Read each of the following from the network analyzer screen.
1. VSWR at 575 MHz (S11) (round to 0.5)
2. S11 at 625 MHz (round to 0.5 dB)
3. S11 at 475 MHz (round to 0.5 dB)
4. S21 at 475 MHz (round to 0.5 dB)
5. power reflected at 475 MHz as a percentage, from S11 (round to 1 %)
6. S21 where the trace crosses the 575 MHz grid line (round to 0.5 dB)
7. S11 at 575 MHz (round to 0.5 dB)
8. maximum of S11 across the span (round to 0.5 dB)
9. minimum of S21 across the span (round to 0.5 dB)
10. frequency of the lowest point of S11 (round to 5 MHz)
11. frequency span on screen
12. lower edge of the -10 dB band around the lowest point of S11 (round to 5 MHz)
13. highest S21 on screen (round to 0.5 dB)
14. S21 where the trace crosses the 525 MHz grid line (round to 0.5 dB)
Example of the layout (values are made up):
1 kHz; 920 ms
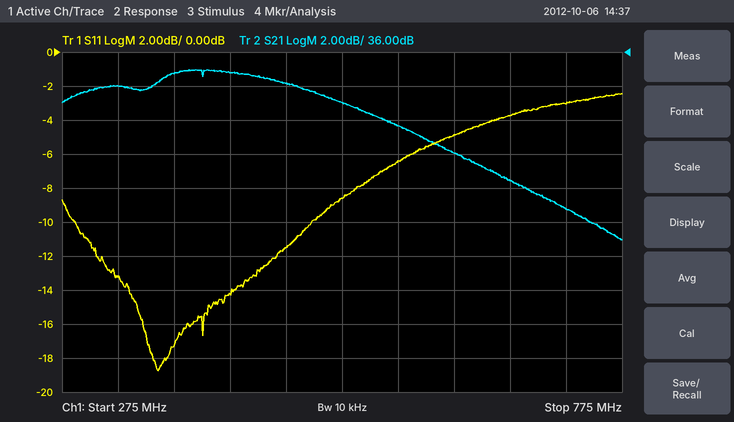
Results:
3.0; -5.0 dB; -11.5 dB; 34.0 dB; 7 %; 31.5 dB; -6.5 dB; -2.5 dB; 25.0 dB; 360 MHz; 500 MHz; 285 MHz; 35.0 dB; 33.0 dB
